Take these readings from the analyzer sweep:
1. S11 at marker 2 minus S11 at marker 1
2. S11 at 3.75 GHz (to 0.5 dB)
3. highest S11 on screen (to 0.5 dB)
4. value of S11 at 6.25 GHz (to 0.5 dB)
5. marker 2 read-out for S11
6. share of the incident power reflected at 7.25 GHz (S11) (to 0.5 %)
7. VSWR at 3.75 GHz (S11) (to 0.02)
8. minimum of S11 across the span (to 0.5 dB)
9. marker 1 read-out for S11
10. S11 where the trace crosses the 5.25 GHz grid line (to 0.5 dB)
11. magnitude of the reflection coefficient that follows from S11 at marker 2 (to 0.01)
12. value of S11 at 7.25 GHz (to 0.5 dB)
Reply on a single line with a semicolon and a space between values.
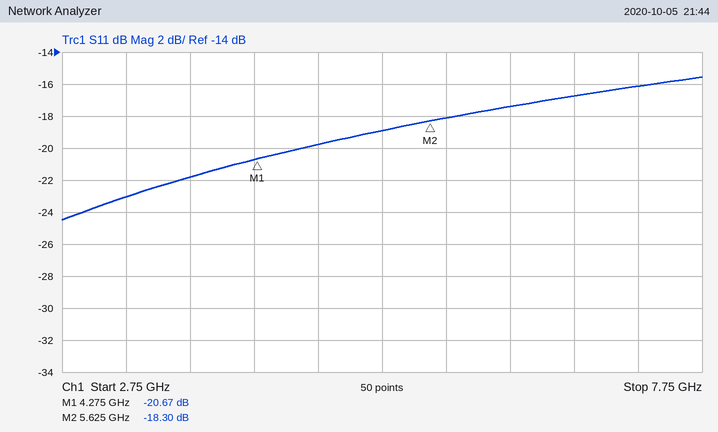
2.37 dB; -22.0 dB; -15.5 dB; -17.5 dB; -18.30 dB; 2.5 %; 1.18; -24.5 dB; -20.67 dB; -19.0 dB; 0.12; -16.0 dB
